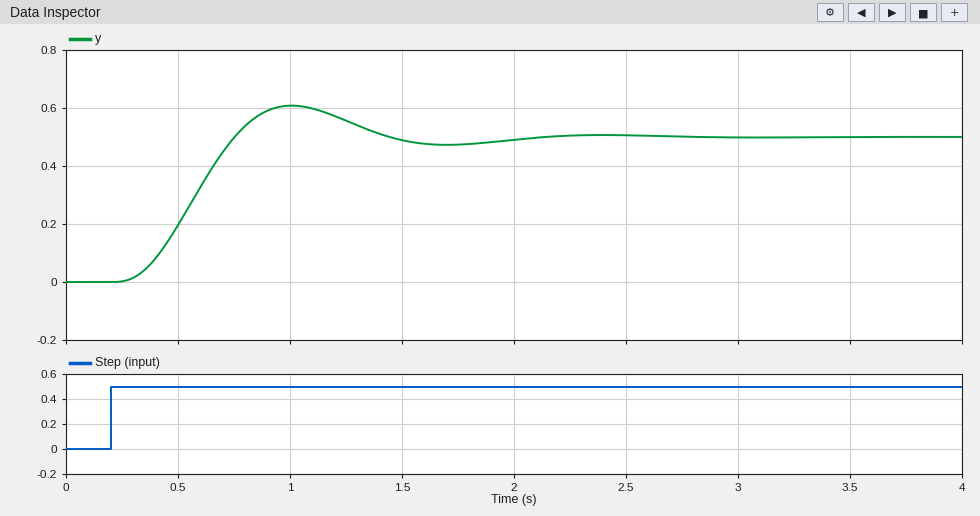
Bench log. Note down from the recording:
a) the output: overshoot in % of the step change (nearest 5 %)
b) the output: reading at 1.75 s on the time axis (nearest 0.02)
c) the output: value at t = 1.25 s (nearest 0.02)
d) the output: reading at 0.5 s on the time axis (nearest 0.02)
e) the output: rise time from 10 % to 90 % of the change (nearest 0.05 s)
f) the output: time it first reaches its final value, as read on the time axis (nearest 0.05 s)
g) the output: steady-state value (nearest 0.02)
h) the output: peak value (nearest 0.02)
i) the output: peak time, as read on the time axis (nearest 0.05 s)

20 %
0.48
0.56
0.20
0.35 s
0.75 s
0.50
0.60
1.00 s
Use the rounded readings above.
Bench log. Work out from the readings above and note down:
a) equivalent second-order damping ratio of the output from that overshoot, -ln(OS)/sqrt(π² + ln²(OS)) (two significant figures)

0.46
